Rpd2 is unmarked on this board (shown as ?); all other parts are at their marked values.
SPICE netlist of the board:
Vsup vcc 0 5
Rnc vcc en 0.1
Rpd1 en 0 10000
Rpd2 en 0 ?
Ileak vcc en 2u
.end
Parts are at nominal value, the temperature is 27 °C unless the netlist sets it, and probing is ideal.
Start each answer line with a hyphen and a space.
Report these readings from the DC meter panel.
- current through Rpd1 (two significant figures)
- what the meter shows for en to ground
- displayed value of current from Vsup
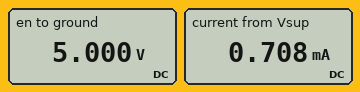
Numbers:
- 500 µA
- 5.000 V
- 0.708 mA
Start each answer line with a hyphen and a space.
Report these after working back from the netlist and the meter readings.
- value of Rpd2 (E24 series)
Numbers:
- 24 kΩ
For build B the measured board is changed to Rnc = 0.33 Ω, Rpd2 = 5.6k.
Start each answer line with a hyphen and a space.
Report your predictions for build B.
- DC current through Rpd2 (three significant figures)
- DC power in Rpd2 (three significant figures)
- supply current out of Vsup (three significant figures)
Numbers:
- 893 µA
- 4.46 mW
- 1.39 mA
